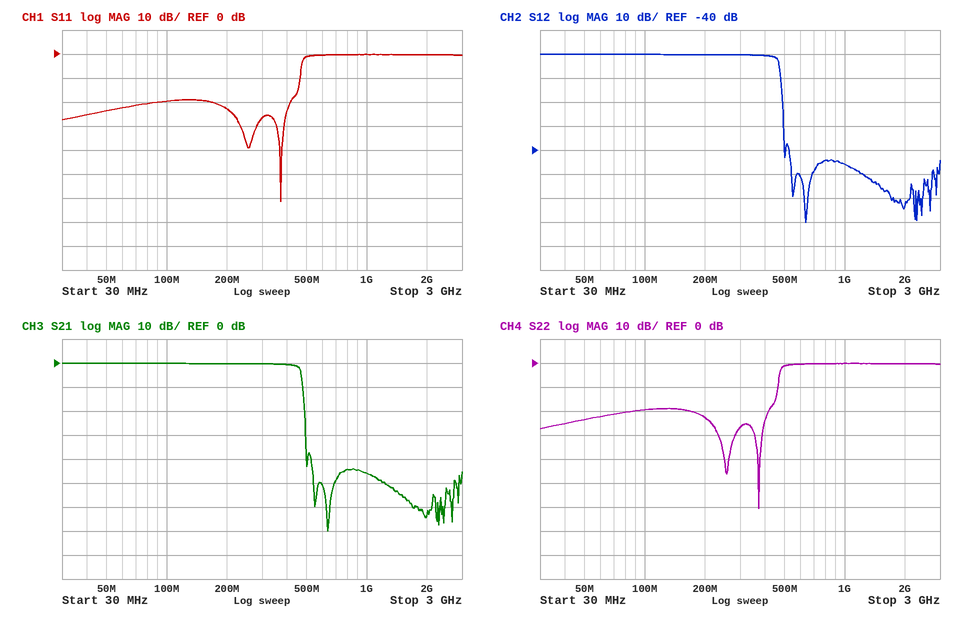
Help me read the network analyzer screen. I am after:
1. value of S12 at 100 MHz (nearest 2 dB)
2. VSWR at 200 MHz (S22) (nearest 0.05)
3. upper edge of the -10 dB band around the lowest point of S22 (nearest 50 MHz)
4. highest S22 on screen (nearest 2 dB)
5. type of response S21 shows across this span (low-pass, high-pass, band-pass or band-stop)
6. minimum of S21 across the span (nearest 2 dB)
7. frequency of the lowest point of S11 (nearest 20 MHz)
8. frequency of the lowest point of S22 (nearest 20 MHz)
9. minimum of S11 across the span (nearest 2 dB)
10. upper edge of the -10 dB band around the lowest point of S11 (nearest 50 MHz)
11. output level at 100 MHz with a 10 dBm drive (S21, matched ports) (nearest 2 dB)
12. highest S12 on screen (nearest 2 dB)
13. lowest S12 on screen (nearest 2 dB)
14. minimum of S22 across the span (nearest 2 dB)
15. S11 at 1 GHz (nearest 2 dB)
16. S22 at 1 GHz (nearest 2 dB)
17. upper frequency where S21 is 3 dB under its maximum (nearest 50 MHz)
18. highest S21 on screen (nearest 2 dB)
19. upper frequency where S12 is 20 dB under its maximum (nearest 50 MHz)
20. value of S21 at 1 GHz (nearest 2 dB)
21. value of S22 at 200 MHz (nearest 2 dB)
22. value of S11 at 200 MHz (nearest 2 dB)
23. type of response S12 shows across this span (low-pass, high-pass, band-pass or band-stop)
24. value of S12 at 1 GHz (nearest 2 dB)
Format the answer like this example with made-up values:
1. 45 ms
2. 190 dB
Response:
1. 0 dB
2. 1.15
3. 450 MHz
4. 0 dB
5. low-pass
6. -70 dB
7. 380 MHz
8. 380 MHz
9. -62 dB
10. 450 MHz
11. 10 dBm
12. 0 dB
13. -70 dB
14. -60 dB
15. 0 dB
16. 0 dB
17. 450 MHz
18. 0 dB
19. 500 MHz
20. -46 dB
21. -22 dB
22. -22 dB
23. low-pass
24. -46 dB
